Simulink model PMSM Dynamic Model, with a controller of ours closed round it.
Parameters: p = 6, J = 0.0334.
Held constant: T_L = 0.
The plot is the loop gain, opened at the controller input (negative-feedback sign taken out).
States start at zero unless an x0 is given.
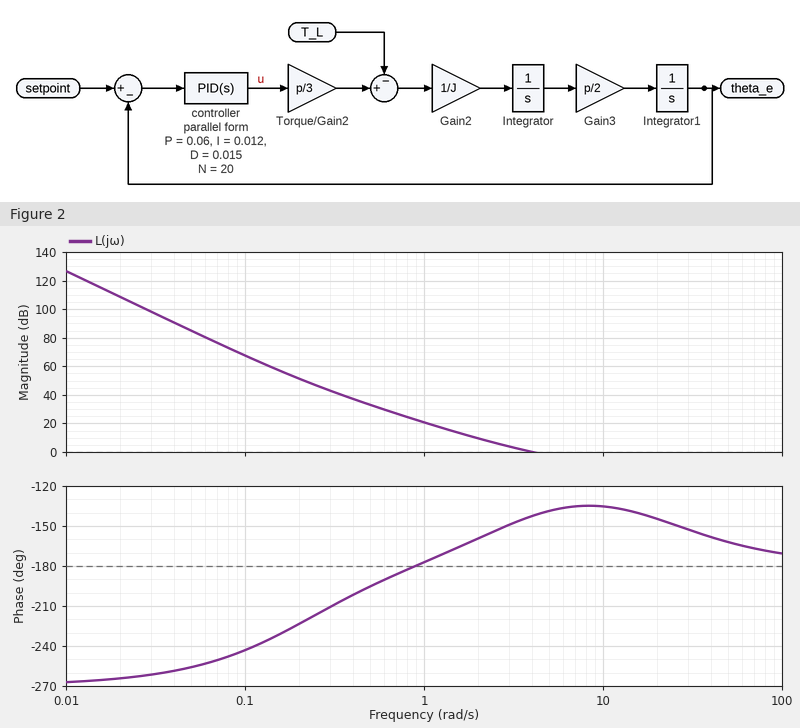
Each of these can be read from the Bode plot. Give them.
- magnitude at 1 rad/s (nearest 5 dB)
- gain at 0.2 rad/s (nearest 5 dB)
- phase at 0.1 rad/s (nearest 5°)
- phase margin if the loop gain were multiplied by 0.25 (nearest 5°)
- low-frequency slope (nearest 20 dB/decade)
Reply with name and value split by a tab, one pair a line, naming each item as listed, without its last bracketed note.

magnitude at 1 rad/s	20 dB
gain at 0.2 rad/s	50 dB
phase at 0.1 rad/s	-245°
phase margin if the loop gain were multiplied by 0.25	15°
low-frequency slope	-60 dB/decade
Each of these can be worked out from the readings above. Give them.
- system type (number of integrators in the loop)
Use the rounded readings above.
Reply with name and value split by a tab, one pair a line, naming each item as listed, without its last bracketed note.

system type	3
